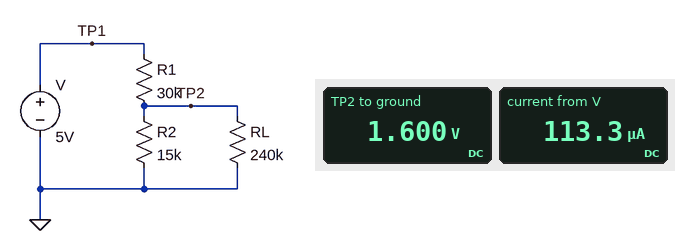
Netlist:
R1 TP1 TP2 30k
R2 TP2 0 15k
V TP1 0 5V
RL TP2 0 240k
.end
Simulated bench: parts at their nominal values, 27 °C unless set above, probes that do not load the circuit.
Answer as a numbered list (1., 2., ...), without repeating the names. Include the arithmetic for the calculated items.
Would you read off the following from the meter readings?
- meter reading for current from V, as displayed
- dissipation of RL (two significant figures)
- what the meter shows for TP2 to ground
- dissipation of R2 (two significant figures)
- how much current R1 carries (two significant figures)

1. 113.3 µA
2. (1.6 V)^2 / 240 kΩ = 11 µW
3. 1.600 V
4. (1.6 V)^2 / 15 kΩ = 170 µW
5. (5 V - 1.6 V) / 30 kΩ = 110 µA
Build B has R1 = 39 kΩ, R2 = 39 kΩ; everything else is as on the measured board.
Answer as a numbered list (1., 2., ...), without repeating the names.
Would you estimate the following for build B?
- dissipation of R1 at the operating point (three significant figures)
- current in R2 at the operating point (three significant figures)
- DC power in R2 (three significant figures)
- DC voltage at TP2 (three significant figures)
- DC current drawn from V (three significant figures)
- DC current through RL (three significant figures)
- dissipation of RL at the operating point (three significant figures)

1. 185 µW
2. 59.3 µA
3. 137 µW
4. 2.31 V
5. 68.9 µA
6. 9.63 µA
7. 22.3 µW
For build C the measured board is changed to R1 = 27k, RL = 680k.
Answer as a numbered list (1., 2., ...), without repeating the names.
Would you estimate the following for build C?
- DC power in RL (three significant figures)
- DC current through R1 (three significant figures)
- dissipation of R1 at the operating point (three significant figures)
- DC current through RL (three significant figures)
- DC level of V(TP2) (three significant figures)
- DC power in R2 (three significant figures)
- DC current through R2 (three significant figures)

1. 4.56 µW
2. 120 µA
3. 389 µW
4. 2.59 µA
5. 1.76 V
6. 207 µW
7. 117 µA
